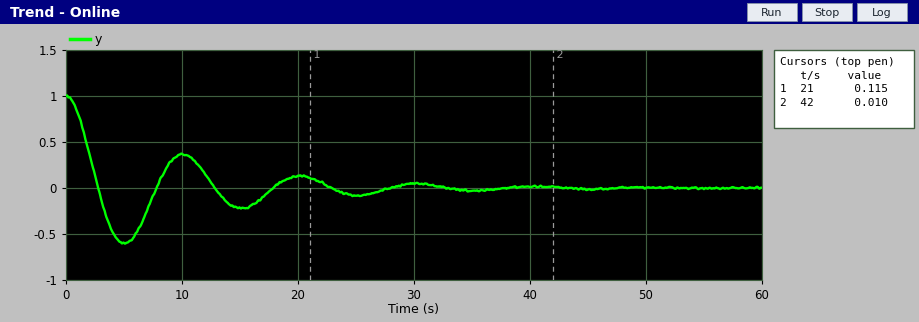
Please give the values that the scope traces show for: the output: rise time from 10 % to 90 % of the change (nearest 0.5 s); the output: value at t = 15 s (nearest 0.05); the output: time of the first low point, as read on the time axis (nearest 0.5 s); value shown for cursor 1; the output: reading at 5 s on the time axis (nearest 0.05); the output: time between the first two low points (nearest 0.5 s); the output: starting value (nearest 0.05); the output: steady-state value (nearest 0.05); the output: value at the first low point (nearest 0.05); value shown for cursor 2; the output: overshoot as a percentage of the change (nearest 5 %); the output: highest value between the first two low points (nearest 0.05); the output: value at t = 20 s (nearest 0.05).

2.0 s
-0.20
5.0 s
0.115
-0.60
10.0 s
1.00
0.00
-0.60
0.010
60 %
0.35
0.15
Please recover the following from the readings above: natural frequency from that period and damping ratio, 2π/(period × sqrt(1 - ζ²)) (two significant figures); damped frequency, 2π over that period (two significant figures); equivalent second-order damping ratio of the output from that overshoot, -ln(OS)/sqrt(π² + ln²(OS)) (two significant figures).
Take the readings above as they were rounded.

0.64 rad/s
0.63 rad/s
0.16
